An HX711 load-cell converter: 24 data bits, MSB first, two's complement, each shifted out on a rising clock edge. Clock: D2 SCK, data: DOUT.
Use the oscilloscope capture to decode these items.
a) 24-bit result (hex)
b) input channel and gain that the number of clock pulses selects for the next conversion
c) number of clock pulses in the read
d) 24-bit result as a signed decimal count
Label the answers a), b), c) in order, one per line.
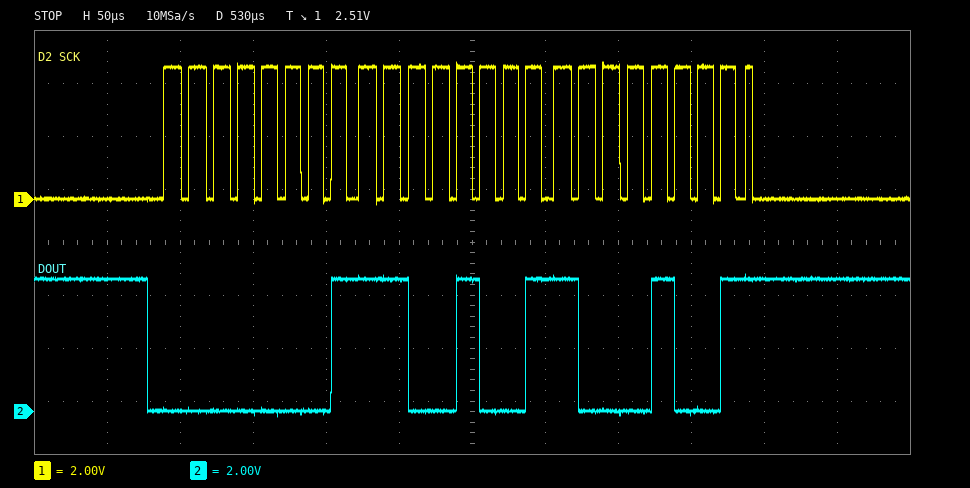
a) 0x01C989
b) channel A, gain 128
c) 25
d) 117129
